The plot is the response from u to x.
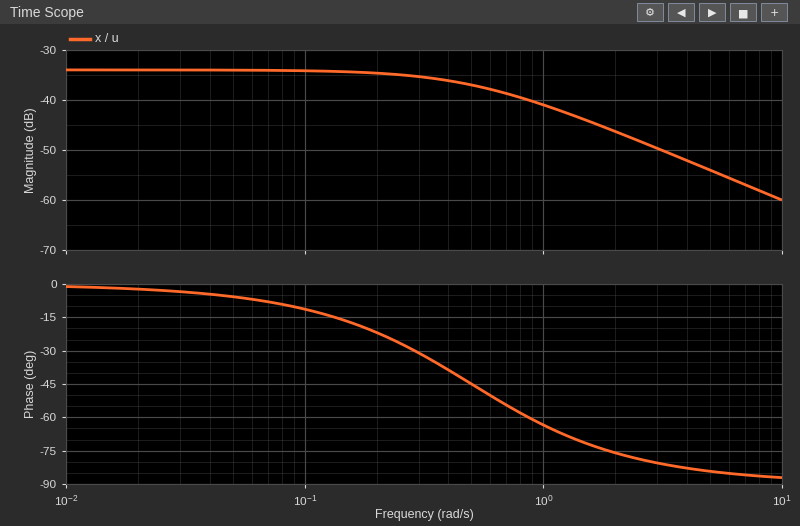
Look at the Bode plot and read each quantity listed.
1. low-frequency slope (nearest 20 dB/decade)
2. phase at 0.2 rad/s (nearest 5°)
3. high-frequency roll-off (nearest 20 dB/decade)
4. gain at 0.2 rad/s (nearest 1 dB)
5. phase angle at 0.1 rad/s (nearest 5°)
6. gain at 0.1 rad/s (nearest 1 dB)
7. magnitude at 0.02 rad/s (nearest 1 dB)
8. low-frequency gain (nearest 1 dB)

0 dB/decade
-20°
-20 dB/decade
-35 dB
-10°
-34 dB
-34 dB
-34 dB
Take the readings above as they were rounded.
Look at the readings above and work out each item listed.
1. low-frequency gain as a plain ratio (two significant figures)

0.020
